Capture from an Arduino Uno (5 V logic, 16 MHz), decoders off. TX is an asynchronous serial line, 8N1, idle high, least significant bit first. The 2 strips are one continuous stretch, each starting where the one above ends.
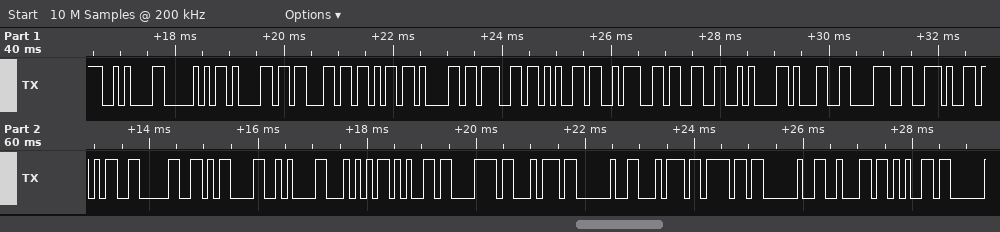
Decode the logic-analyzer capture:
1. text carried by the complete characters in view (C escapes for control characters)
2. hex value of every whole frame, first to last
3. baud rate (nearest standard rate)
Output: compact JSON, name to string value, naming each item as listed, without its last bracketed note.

{"text carried by the complete characters in view": "\"\\nPackage:3\\n18.50\\r\\nText to be\"", "hex value of every whole frame, first to last": "0A 50 61 63 6B 61 67 65 3A 33 0A 31 38 2E 35 30 0D 0A 54 65 78 74 20 74 6F 20 62 65", "baud rate": "9600 baud"}
